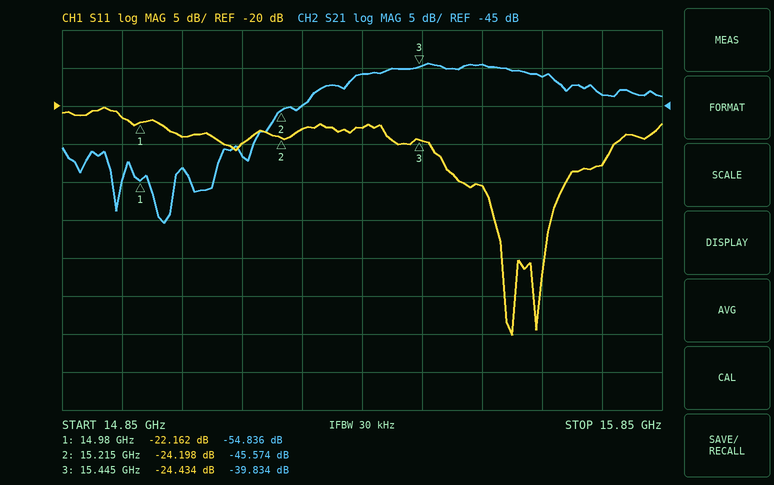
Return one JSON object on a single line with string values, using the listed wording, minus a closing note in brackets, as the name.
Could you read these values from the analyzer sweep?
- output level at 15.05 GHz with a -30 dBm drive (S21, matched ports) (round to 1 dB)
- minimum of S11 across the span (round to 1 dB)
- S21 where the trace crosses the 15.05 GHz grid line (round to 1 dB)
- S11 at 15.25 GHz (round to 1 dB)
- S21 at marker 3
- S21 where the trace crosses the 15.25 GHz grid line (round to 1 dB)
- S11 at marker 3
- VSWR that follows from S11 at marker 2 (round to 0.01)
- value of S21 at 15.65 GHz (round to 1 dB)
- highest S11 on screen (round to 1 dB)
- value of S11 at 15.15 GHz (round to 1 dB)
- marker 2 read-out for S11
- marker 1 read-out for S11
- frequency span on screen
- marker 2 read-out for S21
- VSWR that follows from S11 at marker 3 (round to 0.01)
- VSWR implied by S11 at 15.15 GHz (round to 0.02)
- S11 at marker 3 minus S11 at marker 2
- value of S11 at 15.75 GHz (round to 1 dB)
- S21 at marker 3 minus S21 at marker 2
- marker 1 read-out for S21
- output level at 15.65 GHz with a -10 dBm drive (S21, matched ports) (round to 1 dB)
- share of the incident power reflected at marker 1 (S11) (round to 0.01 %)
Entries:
{"output level at 15.05 GHz with a -30 dBm drive (S21, matched ports)": "-83 dBm", "minimum of S11 across the span": "-50 dB", "S21 where the trace crosses the 15.05 GHz grid line": "-53 dB", "S11 at 15.25 GHz": "-23 dB", "S21 at marker 3": "-39.834 dB", "S21 where the trace crosses the 15.25 GHz grid line": "-45 dB", "S11 at marker 3": "-24.434 dB", "VSWR that follows from S11 at marker 2": "1.13", "value of S21 at 15.65 GHz": "-41 dB", "highest S11 on screen": "-20 dB", "value of S11 at 15.15 GHz": "-25 dB", "marker 2 read-out for S11": "-24.198 dB", "marker 1 read-out for S11": "-22.162 dB", "frequency span on screen": "1 GHz", "marker 2 read-out for S21": "-45.574 dB", "VSWR that follows from S11 at marker 3": "1.13", "VSWR implied by S11 at 15.15 GHz": "1.12", "S11 at marker 3 minus S11 at marker 2": "-0.236 dB", "value of S11 at 15.75 GHz": "-28 dB", "S21 at marker 3 minus S21 at marker 2": "5.740 dB", "marker 1 read-out for S21": "-54.836 dB", "output level at 15.65 GHz with a -10 dBm drive (S21, matched ports)": "-51 dBm", "share of the incident power reflected at marker 1 (S11)": "0.61 %"}
